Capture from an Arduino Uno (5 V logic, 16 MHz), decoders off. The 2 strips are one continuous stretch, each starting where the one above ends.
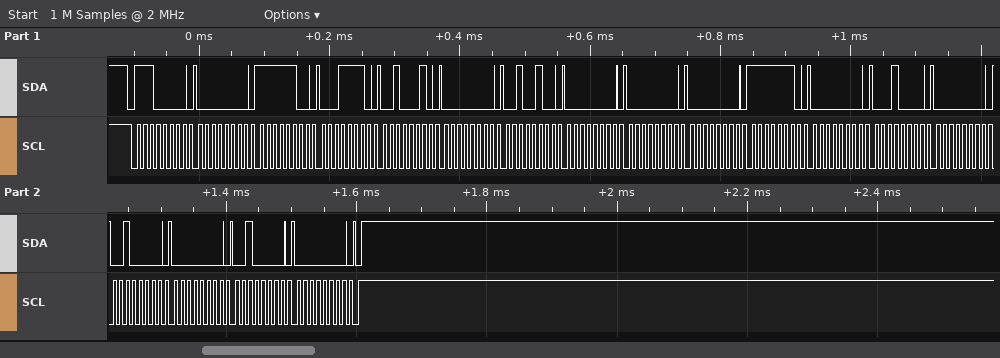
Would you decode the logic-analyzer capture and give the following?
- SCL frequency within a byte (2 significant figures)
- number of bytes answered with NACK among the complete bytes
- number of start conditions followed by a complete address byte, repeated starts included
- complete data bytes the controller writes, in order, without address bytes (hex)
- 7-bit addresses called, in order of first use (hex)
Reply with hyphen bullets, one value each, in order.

- 100 kHz
- 0
- 1
- 00 FC 1E 22 00 24 00 00 00 FE 00 10 00 20 00 20 00
- 0x70
